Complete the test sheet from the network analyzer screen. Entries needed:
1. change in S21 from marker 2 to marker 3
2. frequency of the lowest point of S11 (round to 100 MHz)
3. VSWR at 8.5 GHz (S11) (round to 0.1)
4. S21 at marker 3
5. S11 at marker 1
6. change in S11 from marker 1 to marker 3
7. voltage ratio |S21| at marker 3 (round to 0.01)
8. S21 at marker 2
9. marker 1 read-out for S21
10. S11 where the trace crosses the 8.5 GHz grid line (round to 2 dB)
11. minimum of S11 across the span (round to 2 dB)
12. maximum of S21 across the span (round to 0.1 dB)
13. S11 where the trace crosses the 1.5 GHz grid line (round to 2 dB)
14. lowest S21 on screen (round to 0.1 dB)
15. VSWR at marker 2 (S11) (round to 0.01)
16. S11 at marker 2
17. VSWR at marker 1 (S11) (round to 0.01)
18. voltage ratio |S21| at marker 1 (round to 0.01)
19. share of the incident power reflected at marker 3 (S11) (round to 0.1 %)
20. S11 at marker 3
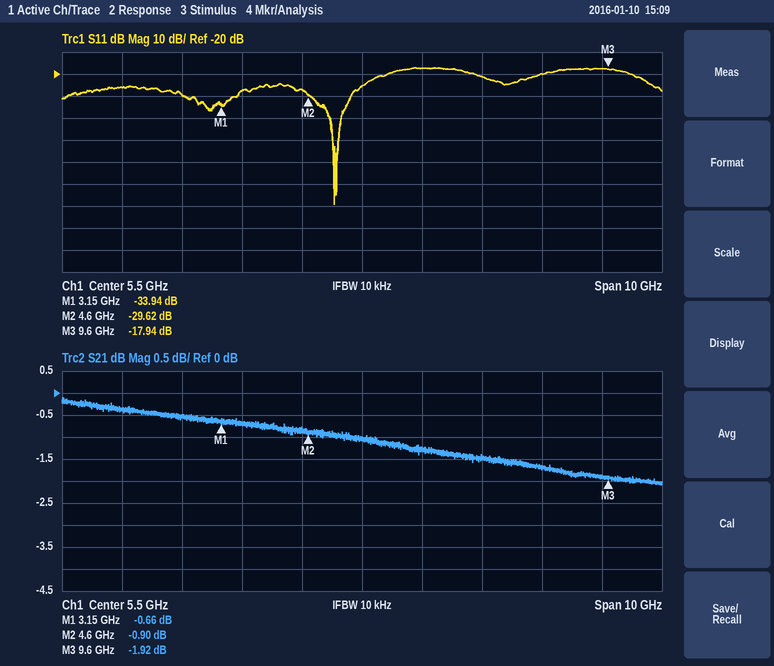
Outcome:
-1.02 dB
5.0 GHz
1.2
-1.92 dB
-33.94 dB
16.00 dB
0.80
-0.90 dB
-0.66 dB
-20 dB
-80 dB
-0.1 dB
-26 dB
-2.1 dB
1.07
-29.62 dB
1.04
0.93
1.6 %
-17.94 dB
